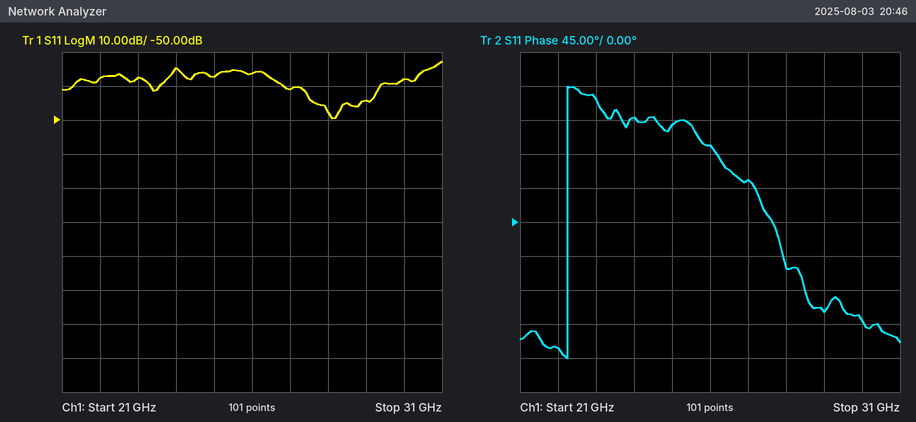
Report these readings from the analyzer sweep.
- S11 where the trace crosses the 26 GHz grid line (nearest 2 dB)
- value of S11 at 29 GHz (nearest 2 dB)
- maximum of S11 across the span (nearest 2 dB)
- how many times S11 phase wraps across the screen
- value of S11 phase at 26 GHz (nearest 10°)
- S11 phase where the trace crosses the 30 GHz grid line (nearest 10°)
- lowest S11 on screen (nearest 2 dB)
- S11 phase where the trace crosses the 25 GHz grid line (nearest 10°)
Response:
-36 dB
-44 dB
-32 dB
1
100°
-130°
-50 dB
130°
